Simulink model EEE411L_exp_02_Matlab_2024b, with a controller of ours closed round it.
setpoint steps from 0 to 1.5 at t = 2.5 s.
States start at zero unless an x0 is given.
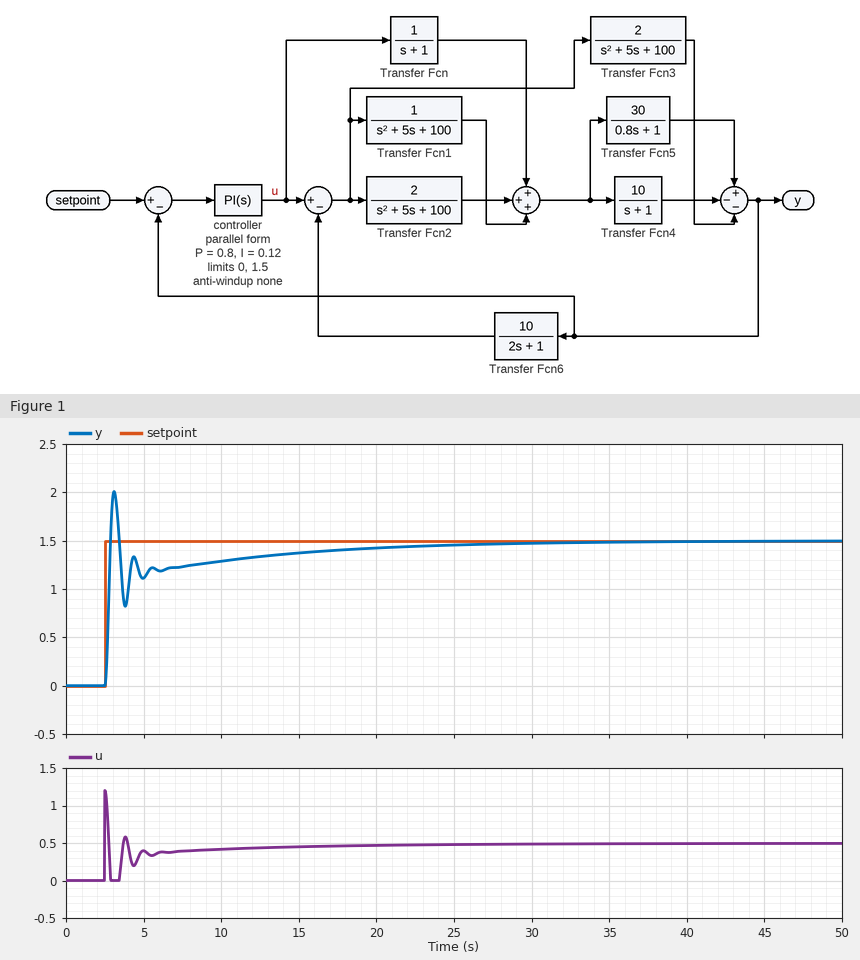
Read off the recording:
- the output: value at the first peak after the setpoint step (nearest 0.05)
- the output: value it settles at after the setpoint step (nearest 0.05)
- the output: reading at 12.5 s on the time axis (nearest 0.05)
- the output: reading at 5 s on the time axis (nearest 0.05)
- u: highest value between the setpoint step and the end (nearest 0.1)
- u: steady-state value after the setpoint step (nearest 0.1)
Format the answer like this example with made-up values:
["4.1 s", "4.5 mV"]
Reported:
["2.00", "1.50", "1.35", "1.10", "1.2", "0.5"]
